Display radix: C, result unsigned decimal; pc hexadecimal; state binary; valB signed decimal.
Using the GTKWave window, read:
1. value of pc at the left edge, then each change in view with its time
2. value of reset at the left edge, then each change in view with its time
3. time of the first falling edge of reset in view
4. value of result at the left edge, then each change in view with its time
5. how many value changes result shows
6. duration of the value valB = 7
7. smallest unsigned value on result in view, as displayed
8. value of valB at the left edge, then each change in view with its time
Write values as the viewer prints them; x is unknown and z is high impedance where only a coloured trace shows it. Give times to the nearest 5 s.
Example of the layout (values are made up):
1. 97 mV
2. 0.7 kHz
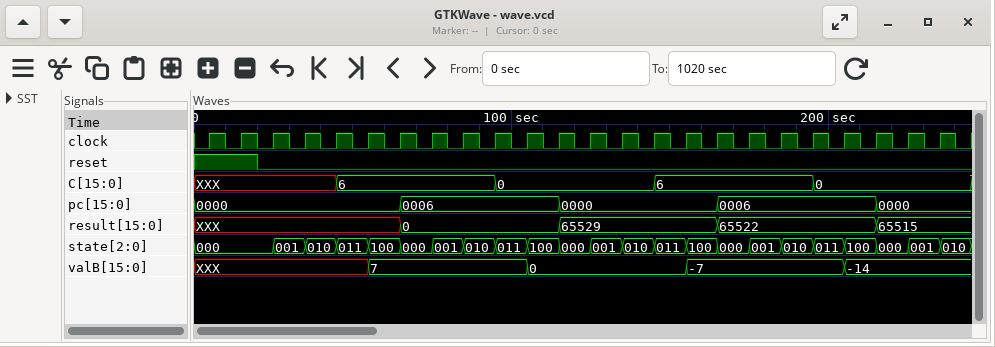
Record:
1. 0000, 0006 at 65 s, 0000 at 115 s, 0006 at 165 s, 0000 at 215 s
2. 1, 0 at 20 s
3. 20 s
4. XXX, 0 at 65 s, 65529 at 115 s, 65522 at 165 s, 65515 at 215 s
5. 4
6. 50 s
7. 0
8. XXX, 7 at 55 s, 0 at 105 s, -7 at 155 s, -14 at 205 s
